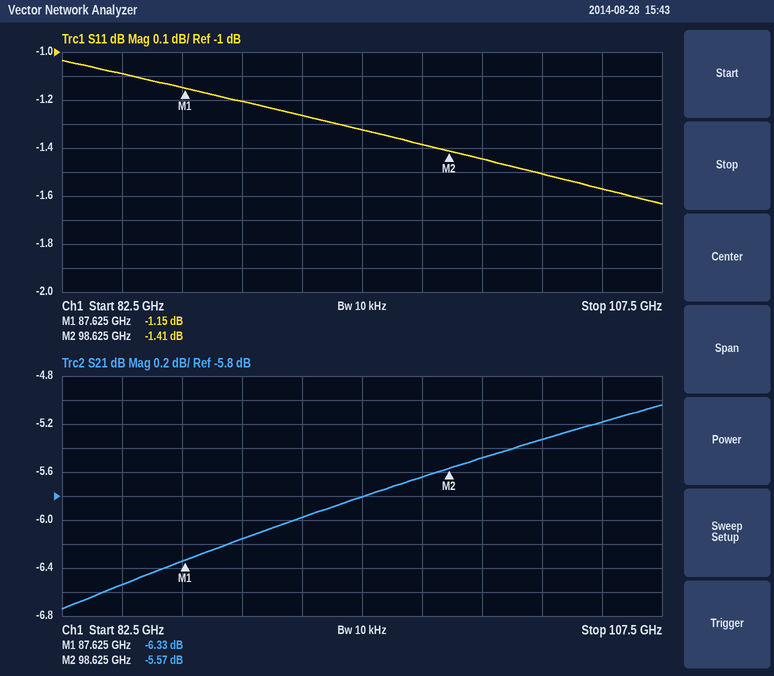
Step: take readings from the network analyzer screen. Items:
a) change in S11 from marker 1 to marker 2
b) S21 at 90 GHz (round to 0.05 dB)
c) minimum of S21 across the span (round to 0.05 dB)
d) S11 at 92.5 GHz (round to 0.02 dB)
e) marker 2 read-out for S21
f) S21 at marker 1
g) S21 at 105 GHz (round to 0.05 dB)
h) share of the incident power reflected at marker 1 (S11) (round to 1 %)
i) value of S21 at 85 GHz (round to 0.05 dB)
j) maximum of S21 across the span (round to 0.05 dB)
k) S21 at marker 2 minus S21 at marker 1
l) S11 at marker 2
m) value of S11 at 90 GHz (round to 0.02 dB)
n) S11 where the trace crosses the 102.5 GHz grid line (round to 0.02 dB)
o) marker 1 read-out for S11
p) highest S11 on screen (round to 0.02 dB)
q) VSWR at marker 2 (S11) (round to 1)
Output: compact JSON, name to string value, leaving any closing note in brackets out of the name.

{"change in S11 from marker 1 to marker 2": "-0.26 dB", "S21 at 90 GHz": "-6.15 dB", "minimum of S21 across the span": "-6.75 dB", "S11 at 92.5 GHz": "-1.26 dB", "marker 2 read-out for S21": "-5.57 dB", "S21 at marker 1": "-6.33 dB", "S21 at 105 GHz": "-5.20 dB", "share of the incident power reflected at marker 1 (S11)": "77 %", "value of S21 at 85 GHz": "-6.55 dB", "maximum of S21 across the span": "-5.05 dB", "S21 at marker 2 minus S21 at marker 1": "0.76 dB", "S11 at marker 2": "-1.41 dB", "value of S11 at 90 GHz": "-1.20 dB", "S11 where the trace crosses the 102.5 GHz grid line": "-1.50 dB", "marker 1 read-out for S11": "-1.15 dB", "highest S11 on screen": "-1.04 dB", "VSWR at marker 2 (S11)": "12"}
